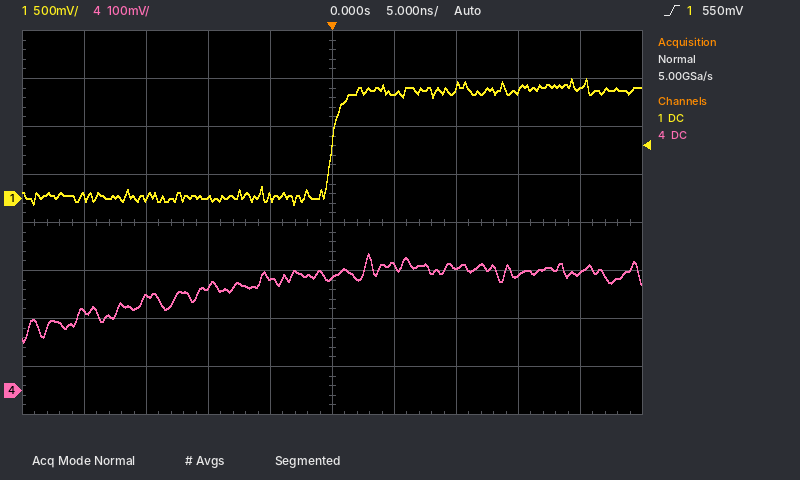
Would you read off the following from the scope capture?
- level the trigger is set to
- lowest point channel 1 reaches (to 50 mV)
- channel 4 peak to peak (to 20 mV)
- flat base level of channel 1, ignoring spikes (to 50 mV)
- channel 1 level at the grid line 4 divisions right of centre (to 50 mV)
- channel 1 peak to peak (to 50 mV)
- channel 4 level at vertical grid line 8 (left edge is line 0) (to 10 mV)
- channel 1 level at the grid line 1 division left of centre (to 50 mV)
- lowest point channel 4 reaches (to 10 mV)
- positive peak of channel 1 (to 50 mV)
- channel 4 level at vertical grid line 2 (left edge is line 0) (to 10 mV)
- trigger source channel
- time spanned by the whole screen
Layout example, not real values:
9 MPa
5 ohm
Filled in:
550 mV
-50 mV
180 mV
0 mV
1.15 V
1.30 V
240 mV
0 mV
100 mV
1.25 V
200 mV
channel 1
50 ns
